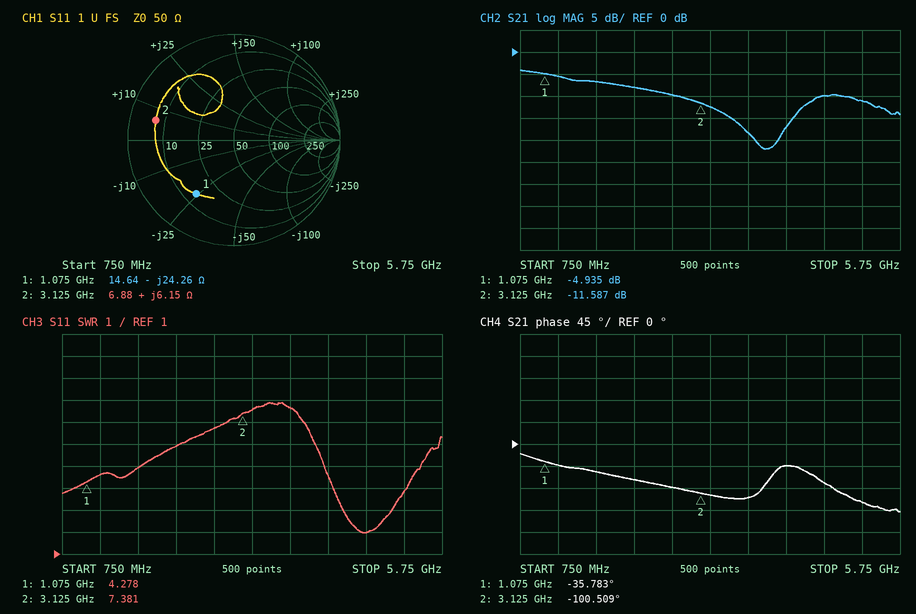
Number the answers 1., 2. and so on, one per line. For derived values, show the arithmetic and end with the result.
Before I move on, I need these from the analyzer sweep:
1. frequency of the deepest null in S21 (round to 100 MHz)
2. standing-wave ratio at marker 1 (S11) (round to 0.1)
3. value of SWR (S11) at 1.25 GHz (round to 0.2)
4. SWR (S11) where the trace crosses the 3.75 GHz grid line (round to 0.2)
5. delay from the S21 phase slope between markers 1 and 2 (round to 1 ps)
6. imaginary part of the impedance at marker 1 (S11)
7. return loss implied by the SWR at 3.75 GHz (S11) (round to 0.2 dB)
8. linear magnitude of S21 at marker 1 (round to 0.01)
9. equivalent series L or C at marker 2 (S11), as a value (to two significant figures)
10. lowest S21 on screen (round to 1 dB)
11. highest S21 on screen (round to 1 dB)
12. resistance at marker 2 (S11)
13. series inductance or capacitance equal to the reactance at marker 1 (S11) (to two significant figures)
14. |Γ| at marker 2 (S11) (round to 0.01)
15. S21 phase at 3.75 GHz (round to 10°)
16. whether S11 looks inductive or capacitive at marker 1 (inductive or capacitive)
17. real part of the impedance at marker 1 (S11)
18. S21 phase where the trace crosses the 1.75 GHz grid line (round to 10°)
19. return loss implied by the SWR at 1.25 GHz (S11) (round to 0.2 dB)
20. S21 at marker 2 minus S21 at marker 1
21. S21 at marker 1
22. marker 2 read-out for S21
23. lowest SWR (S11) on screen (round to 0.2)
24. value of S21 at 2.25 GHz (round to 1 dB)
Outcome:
1. 4.0 GHz
2. 4.3
3. 4.6
4. 7.6
5. −(-100.509° − (-35.783°))/(360° × 2.05 GHz) ≈ 88 ps
6. -24.26 Ω
7. −20 log10((7.6 − 1)/(7.6 + 1)) ≈ 2.30 dB, so 2.2 dB to the nearest 0.2 dB
8. 10^(-4.935/20) ≈ 0.57
9. L = 6.15 Ω/(2π × 3.125 GHz) ≈ 313 pH, so 310 pH to two significant figures
10. -22 dB
11. -4 dB
12. 6.88 Ω
13. C = 1/(2π × 1.075 GHz × 24.26 Ω) ≈ 6.1 pF
14. 0.76
15. -110°
16. capacitive
17. 14.64 Ω
18. -60°
19. −20 log10((4.6 − 1)/(4.6 + 1)) ≈ 3.8 dB
20. -11.587 − (-4.935) = -6.652 dB
21. -4.935 dB
22. -11.587 dB
23. 2.0
24. -8 dB
